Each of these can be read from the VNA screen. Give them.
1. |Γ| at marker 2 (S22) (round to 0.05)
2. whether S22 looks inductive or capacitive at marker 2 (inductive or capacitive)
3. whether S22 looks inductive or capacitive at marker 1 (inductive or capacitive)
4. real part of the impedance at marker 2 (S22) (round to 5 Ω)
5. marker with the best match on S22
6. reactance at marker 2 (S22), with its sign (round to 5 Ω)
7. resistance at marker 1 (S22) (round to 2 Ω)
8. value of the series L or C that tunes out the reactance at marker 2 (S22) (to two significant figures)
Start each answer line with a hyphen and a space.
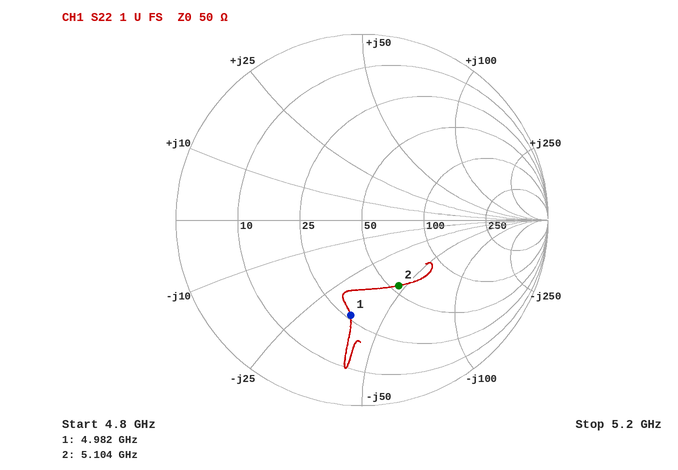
- 0.40
- capacitive
- capacitive
- 55 Ω
- marker 2
- -45 Ω
- 26 Ω
- 1.4 nH
